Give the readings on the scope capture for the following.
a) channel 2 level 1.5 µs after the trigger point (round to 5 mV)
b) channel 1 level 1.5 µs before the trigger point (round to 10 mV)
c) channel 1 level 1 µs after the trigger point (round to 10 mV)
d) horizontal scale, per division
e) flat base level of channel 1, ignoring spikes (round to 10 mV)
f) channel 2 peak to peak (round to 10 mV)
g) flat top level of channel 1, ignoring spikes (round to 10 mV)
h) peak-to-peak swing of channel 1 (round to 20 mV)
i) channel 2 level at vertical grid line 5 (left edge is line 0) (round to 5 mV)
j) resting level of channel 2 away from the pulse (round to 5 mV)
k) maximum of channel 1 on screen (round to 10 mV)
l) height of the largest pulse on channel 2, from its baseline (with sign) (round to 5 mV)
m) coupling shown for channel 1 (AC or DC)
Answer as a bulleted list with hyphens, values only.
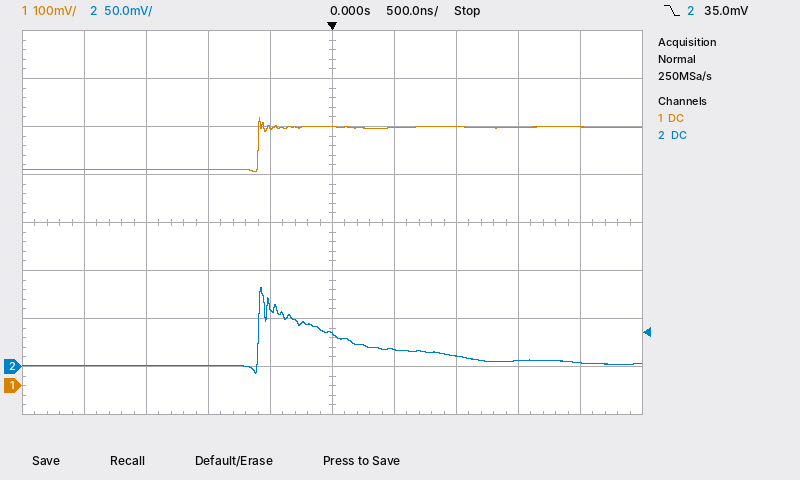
- 5 mV
- 450 mV
- 540 mV
- 500 ns
- 450 mV
- 90 mV
- 540 mV
- 120 mV
- 35 mV
- 0 mV
- 560 mV
- +80 mV
- DC
